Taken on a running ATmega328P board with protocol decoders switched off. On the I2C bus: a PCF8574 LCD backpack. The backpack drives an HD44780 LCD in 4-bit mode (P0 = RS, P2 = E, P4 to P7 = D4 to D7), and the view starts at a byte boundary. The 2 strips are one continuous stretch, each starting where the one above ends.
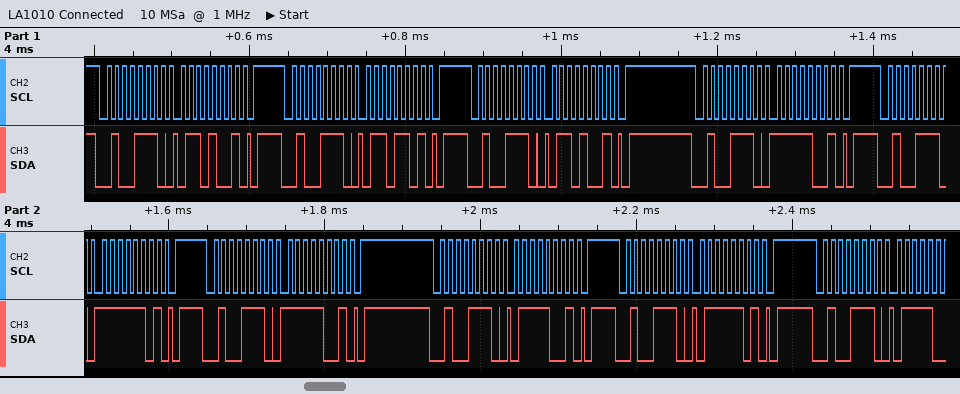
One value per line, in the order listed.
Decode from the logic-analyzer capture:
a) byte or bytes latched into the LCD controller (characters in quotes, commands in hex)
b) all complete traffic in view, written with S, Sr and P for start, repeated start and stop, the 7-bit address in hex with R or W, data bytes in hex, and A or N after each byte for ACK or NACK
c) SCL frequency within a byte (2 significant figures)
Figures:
'o'
S 27W A 69 A P S 27W A 6D A P S 27W A 69 A P S 27W A F9 A P S 27W A FD A P S 27W A F9 A P S 27W A 79 A P S 27W A 7D A P S 27W A
100 kHz
